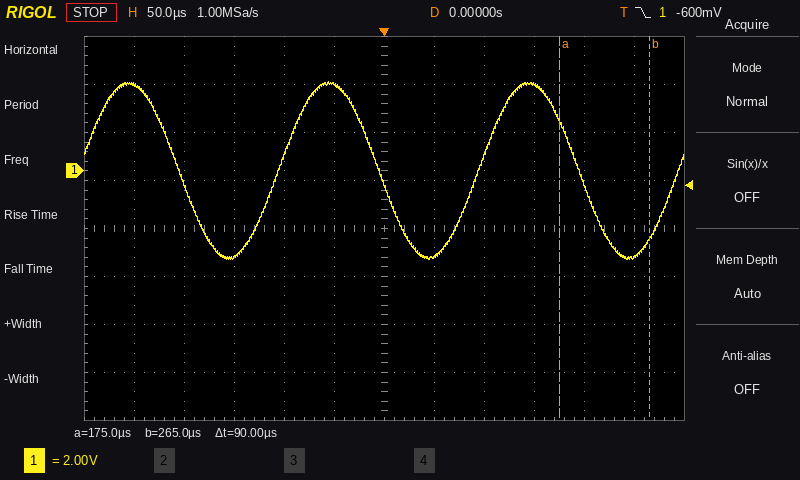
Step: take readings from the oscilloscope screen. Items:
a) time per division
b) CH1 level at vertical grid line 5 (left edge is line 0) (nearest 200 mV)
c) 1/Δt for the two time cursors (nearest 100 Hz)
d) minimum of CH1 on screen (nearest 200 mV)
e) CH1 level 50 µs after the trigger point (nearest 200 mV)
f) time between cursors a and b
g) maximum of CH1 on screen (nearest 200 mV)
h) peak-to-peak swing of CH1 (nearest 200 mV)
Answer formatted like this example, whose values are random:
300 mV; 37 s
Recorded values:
50 µs; 3.6 V; 11.1 kHz; -3.6 V; -3.6 V; 90 µs; 3.8 V; 7.4 V
